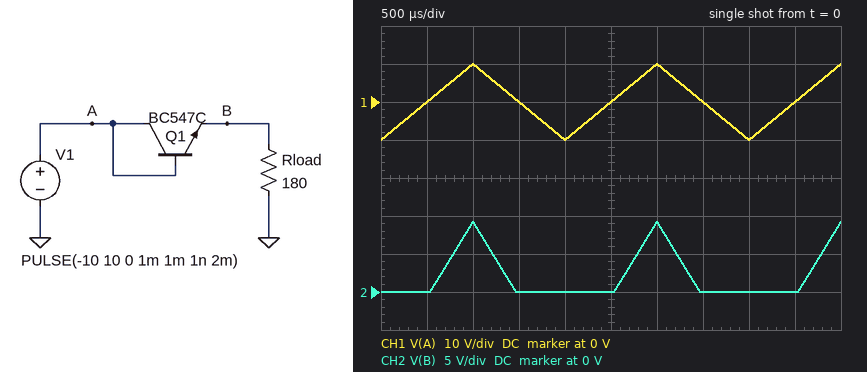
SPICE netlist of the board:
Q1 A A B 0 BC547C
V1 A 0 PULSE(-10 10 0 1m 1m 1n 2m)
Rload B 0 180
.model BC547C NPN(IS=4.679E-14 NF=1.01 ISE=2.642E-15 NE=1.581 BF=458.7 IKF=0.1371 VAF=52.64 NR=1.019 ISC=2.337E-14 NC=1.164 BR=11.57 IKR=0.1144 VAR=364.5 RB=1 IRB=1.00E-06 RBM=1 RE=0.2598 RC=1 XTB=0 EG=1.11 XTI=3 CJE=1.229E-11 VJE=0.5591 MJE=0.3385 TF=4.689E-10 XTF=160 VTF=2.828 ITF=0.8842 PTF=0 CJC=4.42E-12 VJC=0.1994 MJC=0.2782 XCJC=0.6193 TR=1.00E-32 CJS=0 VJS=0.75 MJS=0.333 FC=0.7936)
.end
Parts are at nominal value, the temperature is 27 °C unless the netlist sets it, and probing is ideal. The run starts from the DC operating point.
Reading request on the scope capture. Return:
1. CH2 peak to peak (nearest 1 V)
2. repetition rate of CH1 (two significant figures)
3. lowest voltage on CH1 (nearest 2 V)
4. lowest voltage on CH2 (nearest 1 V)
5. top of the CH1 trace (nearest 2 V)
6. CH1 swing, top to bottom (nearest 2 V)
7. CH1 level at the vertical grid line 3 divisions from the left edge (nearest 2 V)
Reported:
9 V
500 Hz
-10 V
0 V
10 V
20 V
0 V
